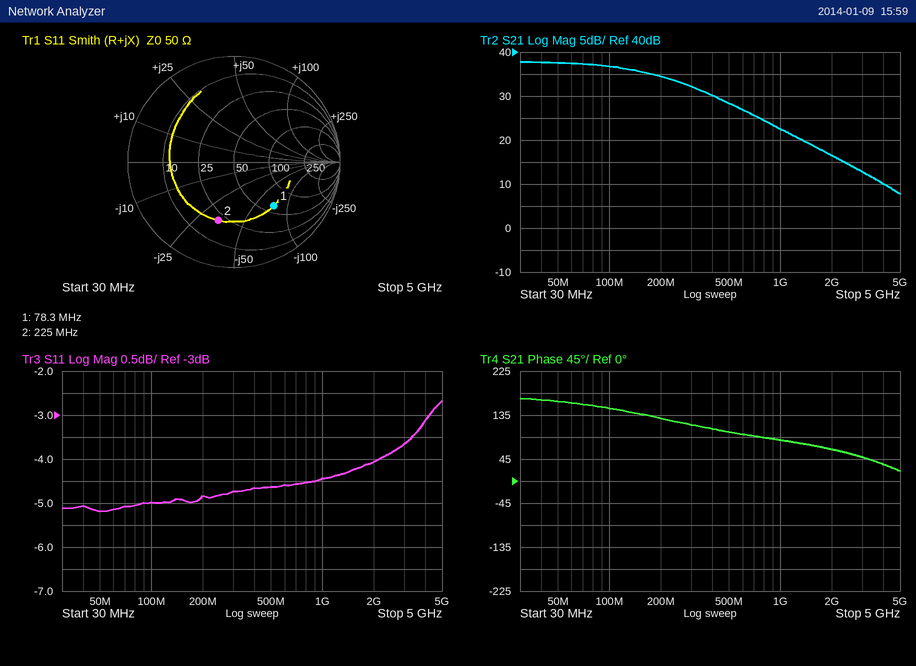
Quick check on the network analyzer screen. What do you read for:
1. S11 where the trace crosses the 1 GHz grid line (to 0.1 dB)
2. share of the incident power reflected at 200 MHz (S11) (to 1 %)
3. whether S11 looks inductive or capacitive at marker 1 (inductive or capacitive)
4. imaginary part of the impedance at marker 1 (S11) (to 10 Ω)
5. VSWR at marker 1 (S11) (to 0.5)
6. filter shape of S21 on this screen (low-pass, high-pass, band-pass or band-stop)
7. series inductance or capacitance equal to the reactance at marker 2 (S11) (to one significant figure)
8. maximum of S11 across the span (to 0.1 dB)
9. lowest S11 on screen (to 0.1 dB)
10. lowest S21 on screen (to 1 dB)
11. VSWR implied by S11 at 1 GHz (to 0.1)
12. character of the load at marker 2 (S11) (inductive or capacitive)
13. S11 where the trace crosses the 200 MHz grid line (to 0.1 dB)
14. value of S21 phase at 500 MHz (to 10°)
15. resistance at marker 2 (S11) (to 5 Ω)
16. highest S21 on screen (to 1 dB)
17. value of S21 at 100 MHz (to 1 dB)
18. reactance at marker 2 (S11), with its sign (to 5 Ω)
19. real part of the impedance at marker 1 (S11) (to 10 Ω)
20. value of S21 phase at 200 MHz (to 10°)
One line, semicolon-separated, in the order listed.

-4.4 dB; 33 %; capacitive; -70 Ω; 3.5; low-pass; 20 pF; -2.7 dB; -5.2 dB; 8 dB; 4.0; capacitive; -4.8 dB; 100°; 20 Ω; 38 dB; 37 dB; -35 Ω; 60 Ω; 130°
